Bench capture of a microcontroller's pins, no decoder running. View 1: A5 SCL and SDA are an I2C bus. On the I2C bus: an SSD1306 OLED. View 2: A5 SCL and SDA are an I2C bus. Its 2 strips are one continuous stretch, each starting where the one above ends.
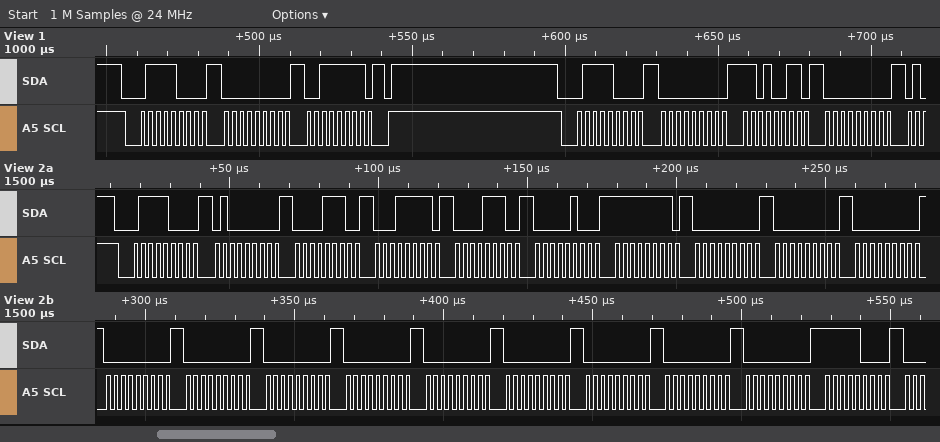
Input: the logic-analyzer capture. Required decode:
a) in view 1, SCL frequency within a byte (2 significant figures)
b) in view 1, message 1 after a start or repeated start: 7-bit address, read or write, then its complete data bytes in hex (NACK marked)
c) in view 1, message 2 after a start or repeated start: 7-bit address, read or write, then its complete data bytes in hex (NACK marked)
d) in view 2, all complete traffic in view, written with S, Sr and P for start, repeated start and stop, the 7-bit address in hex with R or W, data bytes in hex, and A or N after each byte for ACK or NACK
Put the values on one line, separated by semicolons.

400 kHz; 0x3C write: 00 3F; 0x3C write: 00 D3 00; S 3CW A 40 A 0E A 1F A 0E A 04 A FF A 00 A 00 A 00 A 00 A 00 A 00 A 00 A 00 A 00 A 00 A 00 A 00 A F8 A
